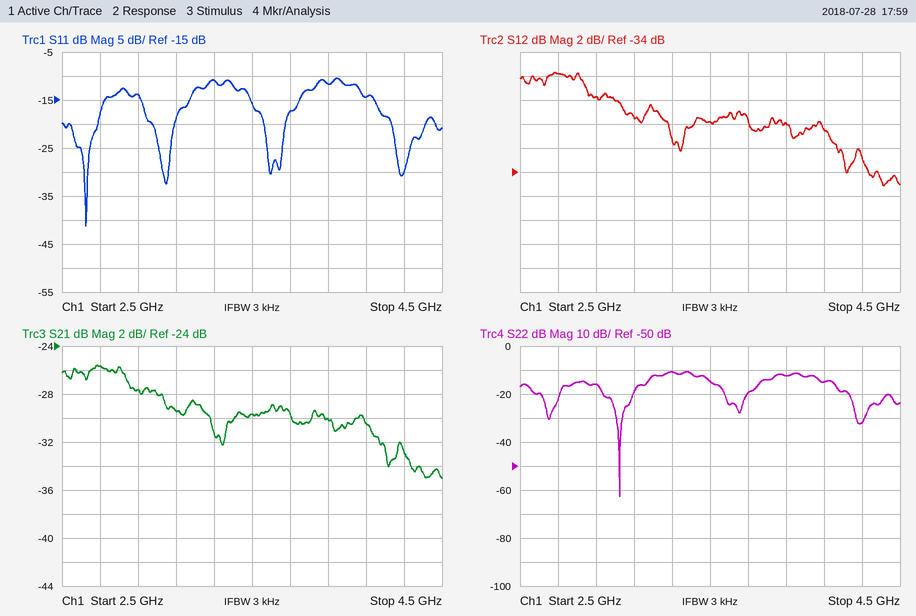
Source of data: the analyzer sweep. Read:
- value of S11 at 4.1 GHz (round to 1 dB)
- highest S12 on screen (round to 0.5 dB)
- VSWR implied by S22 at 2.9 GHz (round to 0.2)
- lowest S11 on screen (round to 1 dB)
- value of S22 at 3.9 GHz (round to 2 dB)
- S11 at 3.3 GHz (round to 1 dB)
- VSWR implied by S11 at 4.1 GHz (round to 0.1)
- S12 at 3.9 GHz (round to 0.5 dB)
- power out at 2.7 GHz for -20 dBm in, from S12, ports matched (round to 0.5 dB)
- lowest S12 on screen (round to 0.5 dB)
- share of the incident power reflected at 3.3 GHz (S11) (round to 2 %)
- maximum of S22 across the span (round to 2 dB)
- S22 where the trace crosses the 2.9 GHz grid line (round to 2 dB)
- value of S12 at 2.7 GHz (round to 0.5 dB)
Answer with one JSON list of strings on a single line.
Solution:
["-14 dB", "-25.5 dB", "1.4", "-41 dB", "-12 dB", "-11 dB", "1.5", "-30.0 dB", "-46.0 dBm", "-35.0 dB", "8 %", "-10 dB", "-16 dB", "-26.0 dB"]
